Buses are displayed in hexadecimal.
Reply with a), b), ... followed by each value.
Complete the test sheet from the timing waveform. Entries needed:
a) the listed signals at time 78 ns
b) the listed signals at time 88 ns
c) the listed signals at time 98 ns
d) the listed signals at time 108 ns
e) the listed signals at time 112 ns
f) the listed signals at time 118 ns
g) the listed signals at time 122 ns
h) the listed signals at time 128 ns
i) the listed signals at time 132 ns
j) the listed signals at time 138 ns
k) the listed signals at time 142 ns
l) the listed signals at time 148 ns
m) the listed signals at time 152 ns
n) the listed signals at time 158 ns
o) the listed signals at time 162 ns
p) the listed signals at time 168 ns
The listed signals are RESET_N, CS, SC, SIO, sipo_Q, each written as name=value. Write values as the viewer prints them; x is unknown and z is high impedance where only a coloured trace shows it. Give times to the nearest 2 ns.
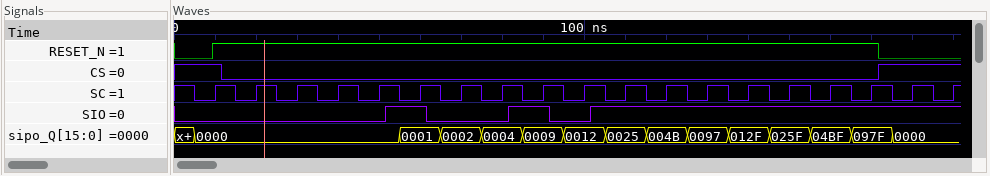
a) RESET_N=1, CS=0, SC=0, SIO=0, sipo_Q=0004
b) RESET_N=1, CS=0, SC=0, SIO=1, sipo_Q=0009
c) RESET_N=1, CS=0, SC=0, SIO=0, sipo_Q=0012
d) RESET_N=1, CS=0, SC=0, SIO=1, sipo_Q=0025
e) RESET_N=1, CS=0, SC=1, SIO=1, sipo_Q=0025
f) RESET_N=1, CS=0, SC=0, SIO=1, sipo_Q=004B
g) RESET_N=1, CS=0, SC=1, SIO=1, sipo_Q=004B
h) RESET_N=1, CS=0, SC=0, SIO=1, sipo_Q=0097
i) RESET_N=1, CS=0, SC=1, SIO=1, sipo_Q=0097
j) RESET_N=1, CS=0, SC=0, SIO=1, sipo_Q=012F
k) RESET_N=1, CS=0, SC=1, SIO=1, sipo_Q=012F
l) RESET_N=1, CS=0, SC=0, SIO=1, sipo_Q=025F
m) RESET_N=1, CS=0, SC=1, SIO=1, sipo_Q=025F
n) RESET_N=1, CS=0, SC=0, SIO=1, sipo_Q=04BF
o) RESET_N=1, CS=0, SC=1, SIO=1, sipo_Q=04BF
p) RESET_N=1, CS=0, SC=0, SIO=1, sipo_Q=097F
